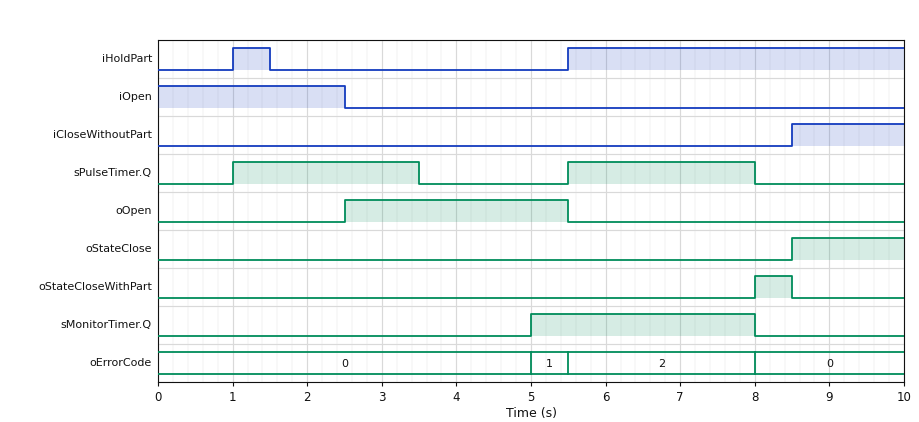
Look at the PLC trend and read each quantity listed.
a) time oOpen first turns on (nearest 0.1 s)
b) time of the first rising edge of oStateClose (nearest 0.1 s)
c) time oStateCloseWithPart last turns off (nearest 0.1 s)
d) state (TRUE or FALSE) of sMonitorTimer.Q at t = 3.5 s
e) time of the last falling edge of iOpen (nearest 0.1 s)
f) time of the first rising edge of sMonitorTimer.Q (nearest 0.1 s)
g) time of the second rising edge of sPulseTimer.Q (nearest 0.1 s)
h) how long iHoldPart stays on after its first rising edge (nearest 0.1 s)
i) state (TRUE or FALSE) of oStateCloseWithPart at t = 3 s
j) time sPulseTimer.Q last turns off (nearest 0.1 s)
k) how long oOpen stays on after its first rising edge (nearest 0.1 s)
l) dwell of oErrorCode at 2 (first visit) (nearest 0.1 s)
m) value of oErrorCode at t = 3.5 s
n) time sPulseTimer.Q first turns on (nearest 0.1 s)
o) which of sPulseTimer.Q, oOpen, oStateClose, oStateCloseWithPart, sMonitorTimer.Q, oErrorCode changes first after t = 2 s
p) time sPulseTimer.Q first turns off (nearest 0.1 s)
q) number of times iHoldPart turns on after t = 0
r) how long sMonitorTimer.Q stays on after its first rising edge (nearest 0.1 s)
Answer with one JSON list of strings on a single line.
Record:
["2.5 s", "8.5 s", "8.5 s", "FALSE", "2.5 s", "5.0 s", "5.5 s", "0.5 s", "FALSE", "8.0 s", "3.0 s", "2.5 s", "0", "1.0 s", "oOpen", "3.5 s", "2", "3.0 s"]
